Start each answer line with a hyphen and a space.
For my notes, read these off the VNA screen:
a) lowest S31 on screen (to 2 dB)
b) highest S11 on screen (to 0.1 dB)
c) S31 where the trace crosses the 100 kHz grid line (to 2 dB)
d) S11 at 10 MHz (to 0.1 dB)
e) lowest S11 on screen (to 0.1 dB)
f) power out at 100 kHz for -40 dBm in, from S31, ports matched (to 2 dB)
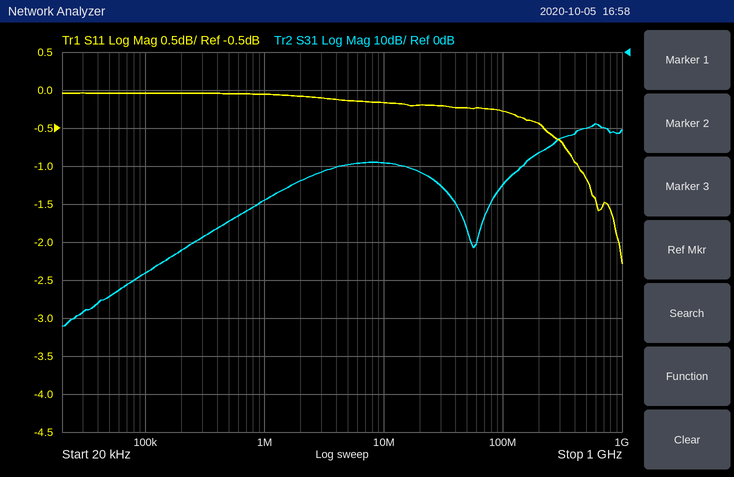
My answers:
- -72 dB
- 0.0 dB
- -58 dB
- -0.2 dB
- -2.3 dB
- -98 dBm
